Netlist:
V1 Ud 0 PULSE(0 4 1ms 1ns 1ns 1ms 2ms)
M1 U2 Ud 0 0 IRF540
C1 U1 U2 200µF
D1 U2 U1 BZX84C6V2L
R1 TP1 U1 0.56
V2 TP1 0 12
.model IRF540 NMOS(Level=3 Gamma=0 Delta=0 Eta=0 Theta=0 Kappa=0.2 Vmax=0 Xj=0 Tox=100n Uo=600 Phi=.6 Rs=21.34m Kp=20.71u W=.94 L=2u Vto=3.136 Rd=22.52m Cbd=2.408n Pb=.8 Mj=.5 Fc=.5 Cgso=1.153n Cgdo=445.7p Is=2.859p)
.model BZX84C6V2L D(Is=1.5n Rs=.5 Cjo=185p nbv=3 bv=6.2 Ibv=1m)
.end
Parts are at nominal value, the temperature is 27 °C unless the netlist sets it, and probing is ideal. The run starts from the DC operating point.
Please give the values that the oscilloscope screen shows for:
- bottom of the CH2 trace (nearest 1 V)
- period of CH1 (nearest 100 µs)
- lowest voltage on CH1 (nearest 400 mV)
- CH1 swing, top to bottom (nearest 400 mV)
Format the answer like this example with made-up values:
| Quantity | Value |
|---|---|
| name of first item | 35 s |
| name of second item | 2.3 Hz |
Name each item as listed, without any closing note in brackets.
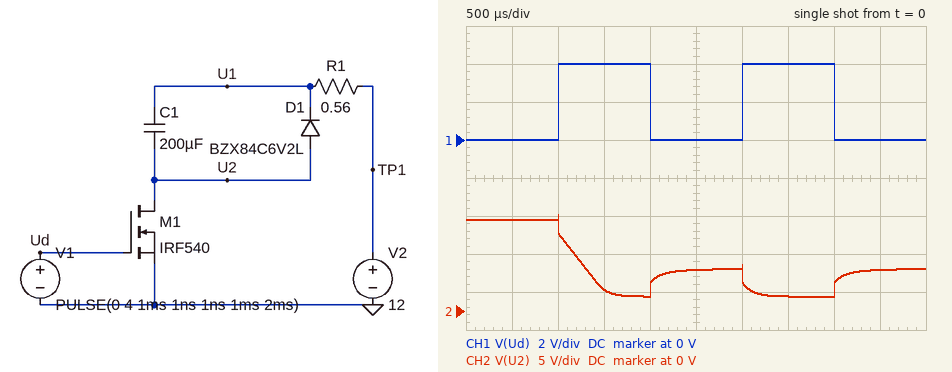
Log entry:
| Quantity | Value |
|---|---|
| bottom of the CH2 trace | 2 V |
| period of CH1 | 2.0 ms |
| lowest voltage on CH1 | 0 V |
| CH1 swing, top to bottom | 4.0 V |
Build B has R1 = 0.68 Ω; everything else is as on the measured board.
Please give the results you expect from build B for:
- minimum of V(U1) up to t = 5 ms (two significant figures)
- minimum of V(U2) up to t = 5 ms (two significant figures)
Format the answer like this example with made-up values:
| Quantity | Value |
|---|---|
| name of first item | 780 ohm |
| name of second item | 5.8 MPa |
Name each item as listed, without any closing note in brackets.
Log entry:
| Quantity | Value |
|---|---|
| minimum of V(U1) up to t = 5 ms | 9.9 V |
| minimum of V(U2) up to t = 5 ms | 1.5 V |
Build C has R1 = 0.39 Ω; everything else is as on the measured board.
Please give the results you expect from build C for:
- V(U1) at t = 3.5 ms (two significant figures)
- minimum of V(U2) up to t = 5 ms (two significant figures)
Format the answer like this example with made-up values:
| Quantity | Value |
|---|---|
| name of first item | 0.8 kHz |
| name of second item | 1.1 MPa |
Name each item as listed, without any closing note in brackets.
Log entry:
| Quantity | Value |
|---|---|
| V(U1) at t = 3.5 ms | 11 V |
| minimum of V(U2) up to t = 5 ms | 2.4 V |
